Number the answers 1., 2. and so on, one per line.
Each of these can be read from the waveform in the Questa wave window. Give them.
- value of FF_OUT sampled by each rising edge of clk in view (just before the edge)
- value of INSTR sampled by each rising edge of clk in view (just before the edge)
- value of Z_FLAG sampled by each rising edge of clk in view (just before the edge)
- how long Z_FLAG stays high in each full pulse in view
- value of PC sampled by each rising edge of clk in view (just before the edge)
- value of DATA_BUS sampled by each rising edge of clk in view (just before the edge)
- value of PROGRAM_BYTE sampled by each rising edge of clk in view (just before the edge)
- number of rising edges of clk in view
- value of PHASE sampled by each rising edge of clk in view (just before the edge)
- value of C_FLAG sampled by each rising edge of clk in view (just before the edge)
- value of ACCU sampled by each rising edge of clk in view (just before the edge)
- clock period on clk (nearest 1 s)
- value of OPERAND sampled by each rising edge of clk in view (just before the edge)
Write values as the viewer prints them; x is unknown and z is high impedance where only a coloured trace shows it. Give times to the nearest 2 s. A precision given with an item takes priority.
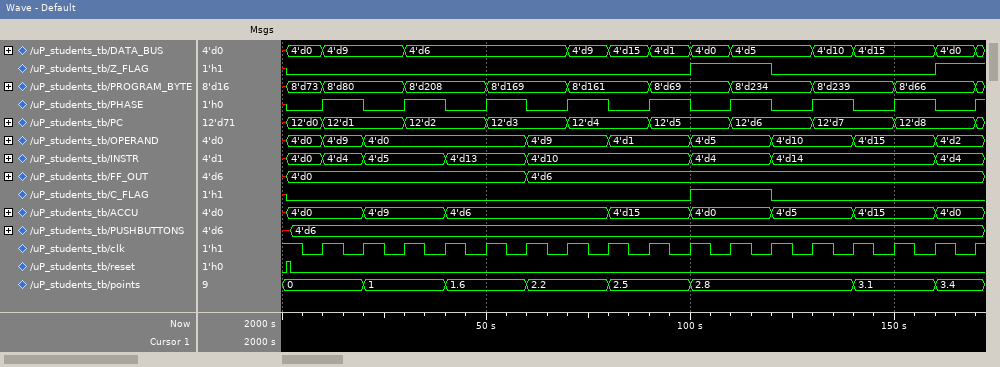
1. 4'd0, 4'd0, 4'd0, 4'd0, 4'd0, 4'd0, 4'd6, 4'd6, 4'd6, 4'd6, 4'd6, 4'd6, 4'd6, 4'd6, 4'd6, 4'd6, 4'd6
2. 4'd0, 4'd4, 4'd5, 4'd5, 4'd13, 4'd13, 4'd10, 4'd10, 4'd10, 4'd10, 4'd4, 4'd4, 4'd14, 4'd14, 4'd14, 4'd14, 4'd4
3. 0 0 0 0 0 0 0 0 0 0 1 1 0 0 0 0 1
4. 20 s
5. 12'd0, 12'd1, 12'd1, 12'd2, 12'd2, 12'd3, 12'd3, 12'd4, 12'd4, 12'd5, 12'd5, 12'd6, 12'd6, 12'd7, 12'd7, 12'd8, 12'd8
6. 4'd0, 4'd9, 4'd9, 4'd6, 4'd6, 4'd6, 4'd6, 4'd9, 4'd15, 4'd1, 4'd0, 4'd5, 4'd5, 4'd10, 4'd15, 4'd15, 4'd0
7. 8'd73, 8'd80, 8'd80, 8'd208, 8'd208, 8'd169, 8'd169, 8'd161, 8'd161, 8'd69, 8'd69, 8'd234, 8'd234, 8'd239, 8'd239, 8'd66, 8'd66
8. 17
9. 0 1 0 1 0 1 0 1 0 1 0 1 0 1 0 1 0
10. 0 0 0 0 0 0 0 0 0 0 1 1 0 0 0 0 0
11. 4'd0, 4'd0, 4'd9, 4'd9, 4'd6, 4'd6, 4'd6, 4'd6, 4'd15, 4'd15, 4'd0, 4'd0, 4'd5, 4'd5, 4'd15, 4'd15, 4'd0
12. 10 s
13. 4'd0, 4'd9, 4'd0, 4'd0, 4'd0, 4'd0, 4'd9, 4'd9, 4'd1, 4'd1, 4'd5, 4'd5, 4'd10, 4'd10, 4'd15, 4'd15, 4'd2
